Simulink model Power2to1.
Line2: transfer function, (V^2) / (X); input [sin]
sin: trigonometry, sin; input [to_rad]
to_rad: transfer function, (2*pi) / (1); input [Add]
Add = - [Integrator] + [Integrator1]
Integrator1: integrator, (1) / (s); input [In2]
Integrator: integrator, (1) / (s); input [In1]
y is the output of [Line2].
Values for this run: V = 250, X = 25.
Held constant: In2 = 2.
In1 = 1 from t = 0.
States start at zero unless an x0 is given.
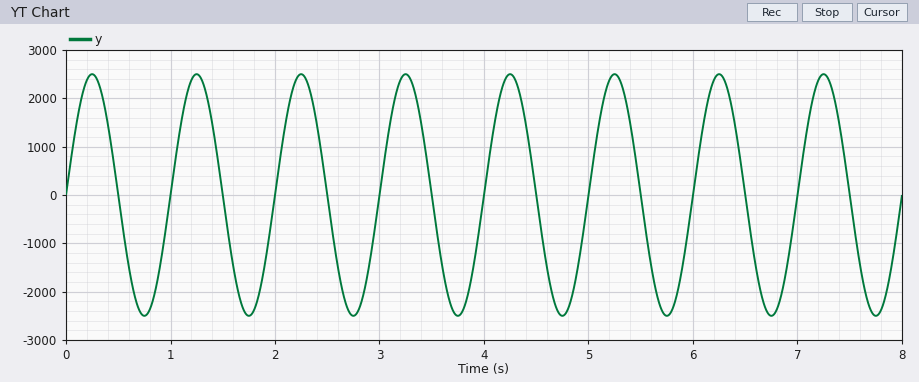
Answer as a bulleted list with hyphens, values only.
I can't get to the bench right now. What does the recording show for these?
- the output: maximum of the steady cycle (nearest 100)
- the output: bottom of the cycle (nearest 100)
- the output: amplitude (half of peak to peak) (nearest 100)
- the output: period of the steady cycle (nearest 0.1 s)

- 2500
- -2500
- 2500
- 1.0 s
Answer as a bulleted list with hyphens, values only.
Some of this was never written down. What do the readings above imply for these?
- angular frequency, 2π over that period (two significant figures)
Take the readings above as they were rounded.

- 6.3 rad/s
